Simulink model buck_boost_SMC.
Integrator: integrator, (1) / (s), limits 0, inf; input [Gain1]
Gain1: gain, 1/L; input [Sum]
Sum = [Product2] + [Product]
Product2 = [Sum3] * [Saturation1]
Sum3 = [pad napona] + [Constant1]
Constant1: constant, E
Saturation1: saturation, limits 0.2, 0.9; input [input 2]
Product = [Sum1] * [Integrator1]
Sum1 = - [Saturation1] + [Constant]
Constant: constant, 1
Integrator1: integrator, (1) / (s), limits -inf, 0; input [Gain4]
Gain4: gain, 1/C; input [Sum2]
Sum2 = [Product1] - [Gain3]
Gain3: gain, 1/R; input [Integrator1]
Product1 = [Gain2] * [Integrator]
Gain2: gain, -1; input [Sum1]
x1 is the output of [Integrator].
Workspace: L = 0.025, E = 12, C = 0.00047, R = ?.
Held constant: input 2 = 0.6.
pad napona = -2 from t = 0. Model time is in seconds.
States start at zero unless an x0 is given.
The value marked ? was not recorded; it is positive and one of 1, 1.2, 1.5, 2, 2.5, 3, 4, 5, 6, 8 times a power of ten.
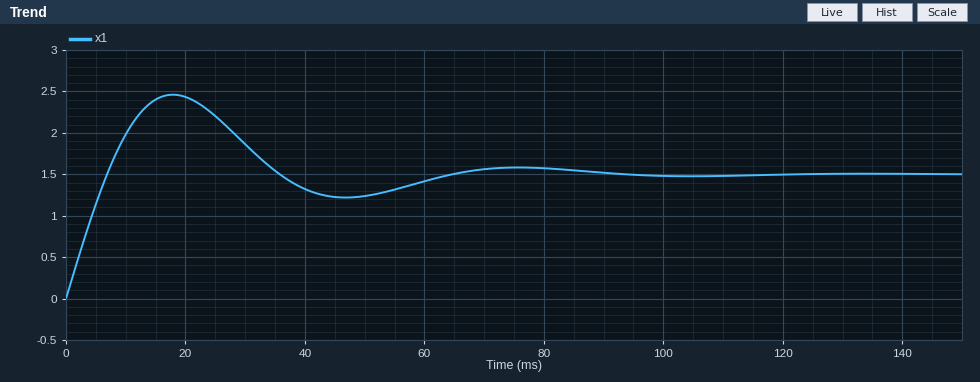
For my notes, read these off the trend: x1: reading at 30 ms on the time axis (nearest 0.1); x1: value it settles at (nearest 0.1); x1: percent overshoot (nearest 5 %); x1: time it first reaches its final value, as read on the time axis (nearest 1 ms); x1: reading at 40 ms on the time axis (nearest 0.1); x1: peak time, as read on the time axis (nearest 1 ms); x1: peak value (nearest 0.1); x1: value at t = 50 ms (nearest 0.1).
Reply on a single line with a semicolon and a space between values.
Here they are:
1.9; 1.5; 65 %; 7 ms; 1.3; 18 ms; 2.5; 1.2
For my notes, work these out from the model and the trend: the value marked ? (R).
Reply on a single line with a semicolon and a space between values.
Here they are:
25
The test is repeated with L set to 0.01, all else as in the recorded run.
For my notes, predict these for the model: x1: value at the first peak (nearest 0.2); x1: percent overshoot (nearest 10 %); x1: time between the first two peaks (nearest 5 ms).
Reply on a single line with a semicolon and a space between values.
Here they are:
3.6; 140 %; 35 ms
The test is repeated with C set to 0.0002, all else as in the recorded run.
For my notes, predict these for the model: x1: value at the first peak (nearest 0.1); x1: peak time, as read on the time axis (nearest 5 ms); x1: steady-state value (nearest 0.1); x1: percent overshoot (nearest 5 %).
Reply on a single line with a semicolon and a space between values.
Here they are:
1.8; 15 ms; 1.5; 20 %
